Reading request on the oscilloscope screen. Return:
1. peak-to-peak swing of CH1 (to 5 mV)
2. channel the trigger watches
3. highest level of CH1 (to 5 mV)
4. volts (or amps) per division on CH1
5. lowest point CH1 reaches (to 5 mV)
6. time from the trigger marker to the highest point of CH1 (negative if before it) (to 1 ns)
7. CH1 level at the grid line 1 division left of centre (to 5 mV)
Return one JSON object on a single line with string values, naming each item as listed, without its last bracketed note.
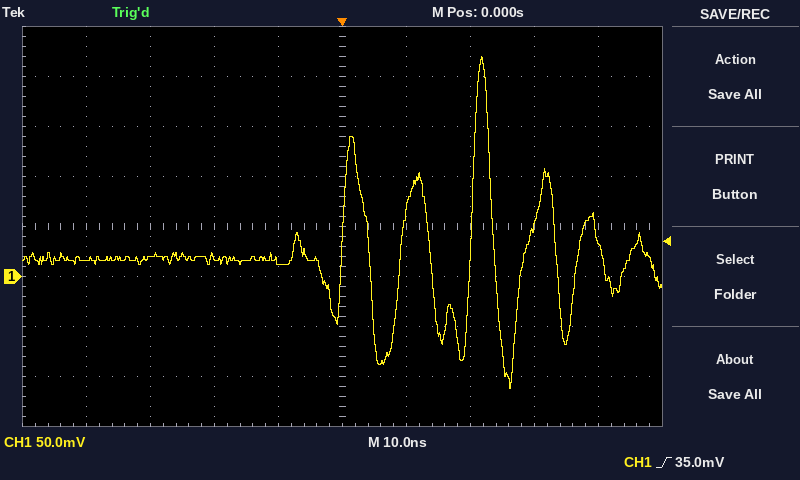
{"peak-to-peak swing of CH1": "330 mV", "channel the trigger watches": "CH1", "highest level of CH1": "220 mV", "volts (or amps) per division on CH1": "50 mV", "lowest point CH1 reaches": "-110 mV", "time from the trigger marker to the highest point of CH1 (negative if before it)": "+22 ns", "CH1 level at the grid line 1 division left of centre": "15 mV"}
